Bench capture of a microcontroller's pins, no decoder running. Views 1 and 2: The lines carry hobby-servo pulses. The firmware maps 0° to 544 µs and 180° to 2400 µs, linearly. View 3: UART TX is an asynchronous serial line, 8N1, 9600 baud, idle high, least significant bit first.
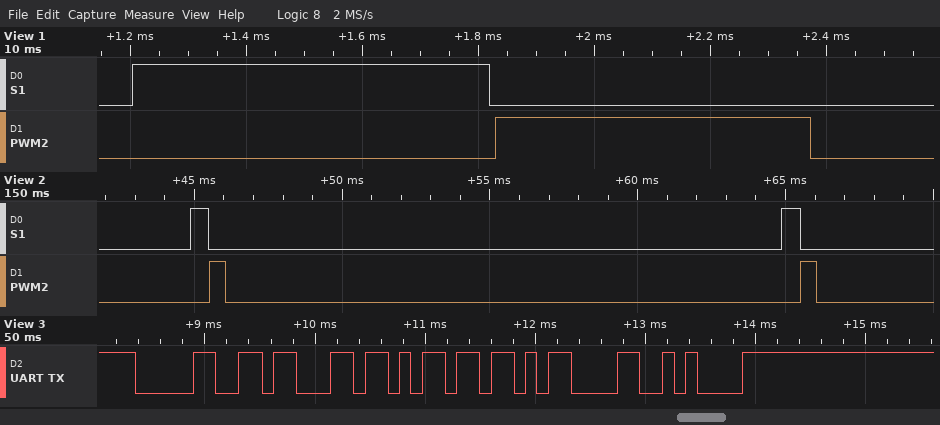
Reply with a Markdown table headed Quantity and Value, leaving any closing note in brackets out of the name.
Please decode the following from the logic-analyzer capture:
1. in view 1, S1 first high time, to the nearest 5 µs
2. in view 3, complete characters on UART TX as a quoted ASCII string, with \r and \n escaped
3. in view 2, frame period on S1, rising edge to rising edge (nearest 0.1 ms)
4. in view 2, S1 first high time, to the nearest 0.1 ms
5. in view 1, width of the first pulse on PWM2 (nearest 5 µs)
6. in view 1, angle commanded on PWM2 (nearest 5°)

| Quantity | Value |
|---|---|
| in view 1, S1 first high time, to the nearest 5 µs | 615 µs |
| in view 3, complete characters on UART TX as a quoted ASCII string, with \r and \n escaped | "0cm\r\n" |
| in view 2, frame period on S1, rising edge to rising edge | 20.0 ms |
| in view 2, S1 first high time, to the nearest 0.1 ms | 0.6 ms |
| in view 1, width of the first pulse on PWM2 | 545 µs |
| in view 1, angle commanded on PWM2 | 0° |
